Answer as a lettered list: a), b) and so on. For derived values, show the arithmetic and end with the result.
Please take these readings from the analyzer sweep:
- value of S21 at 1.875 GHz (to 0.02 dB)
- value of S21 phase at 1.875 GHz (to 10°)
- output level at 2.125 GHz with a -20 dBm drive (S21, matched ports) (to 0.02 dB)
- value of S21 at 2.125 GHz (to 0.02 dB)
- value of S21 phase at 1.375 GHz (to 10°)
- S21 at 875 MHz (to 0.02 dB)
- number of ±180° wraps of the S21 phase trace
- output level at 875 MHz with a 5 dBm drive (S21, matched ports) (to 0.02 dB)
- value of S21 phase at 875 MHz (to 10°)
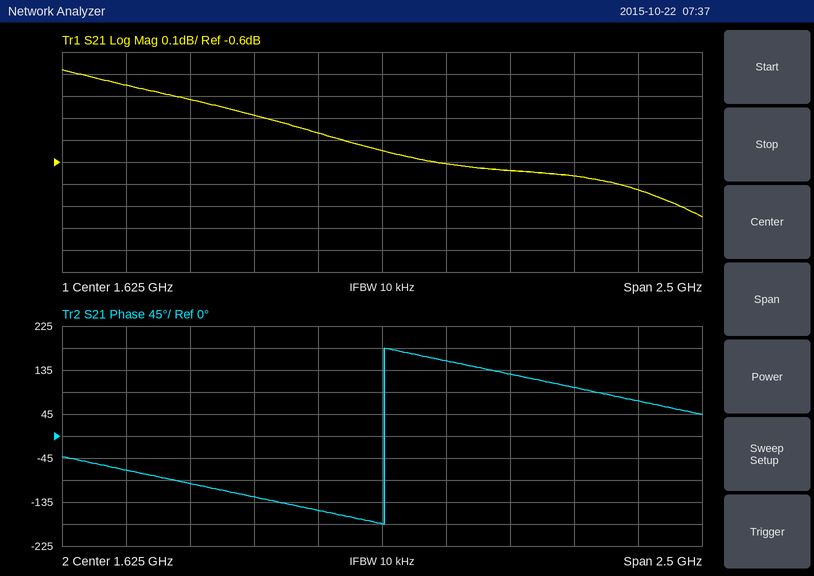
a) -0.60 dB
b) 150°
c) -20 dBm + (-0.64 dB) = -20.64 dBm
d) -0.64 dB
e) -150°
f) -0.32 dB
g) 1
h) 5 dBm + (-0.32 dB) = 4.68 dBm
i) -100°
